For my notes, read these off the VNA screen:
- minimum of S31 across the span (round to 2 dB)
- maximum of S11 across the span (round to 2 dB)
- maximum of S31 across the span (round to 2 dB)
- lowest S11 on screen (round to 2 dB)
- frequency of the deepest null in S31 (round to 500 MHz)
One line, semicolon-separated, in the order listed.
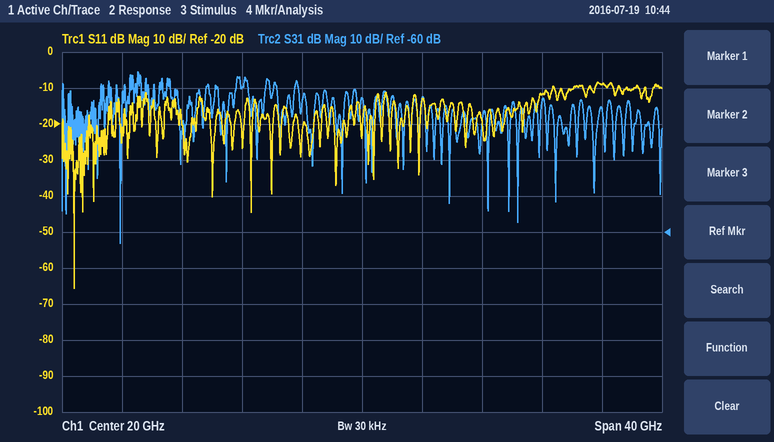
-64 dB; -8 dB; -16 dB; -66 dB; 4.0 GHz
